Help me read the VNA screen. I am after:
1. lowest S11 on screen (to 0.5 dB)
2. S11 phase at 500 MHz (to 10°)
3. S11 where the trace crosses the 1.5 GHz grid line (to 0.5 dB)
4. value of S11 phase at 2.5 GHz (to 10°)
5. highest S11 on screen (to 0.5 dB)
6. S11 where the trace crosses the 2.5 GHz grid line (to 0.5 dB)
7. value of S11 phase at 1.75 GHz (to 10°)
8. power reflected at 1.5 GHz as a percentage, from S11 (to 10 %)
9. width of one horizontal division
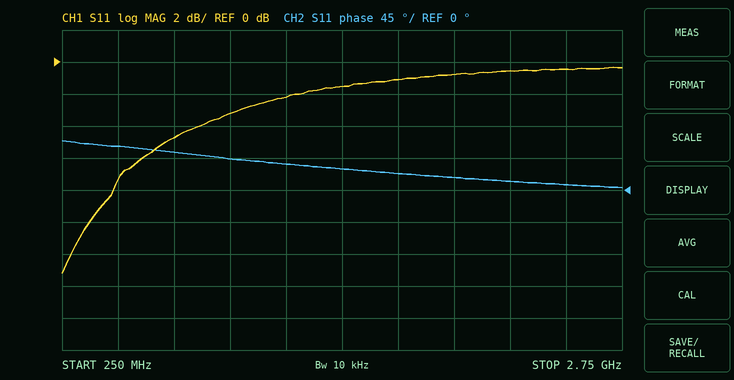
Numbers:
-13.0 dB
60°
-1.5 dB
10°
-0.5 dB
-0.5 dB
20°
70 %
250 MHz
